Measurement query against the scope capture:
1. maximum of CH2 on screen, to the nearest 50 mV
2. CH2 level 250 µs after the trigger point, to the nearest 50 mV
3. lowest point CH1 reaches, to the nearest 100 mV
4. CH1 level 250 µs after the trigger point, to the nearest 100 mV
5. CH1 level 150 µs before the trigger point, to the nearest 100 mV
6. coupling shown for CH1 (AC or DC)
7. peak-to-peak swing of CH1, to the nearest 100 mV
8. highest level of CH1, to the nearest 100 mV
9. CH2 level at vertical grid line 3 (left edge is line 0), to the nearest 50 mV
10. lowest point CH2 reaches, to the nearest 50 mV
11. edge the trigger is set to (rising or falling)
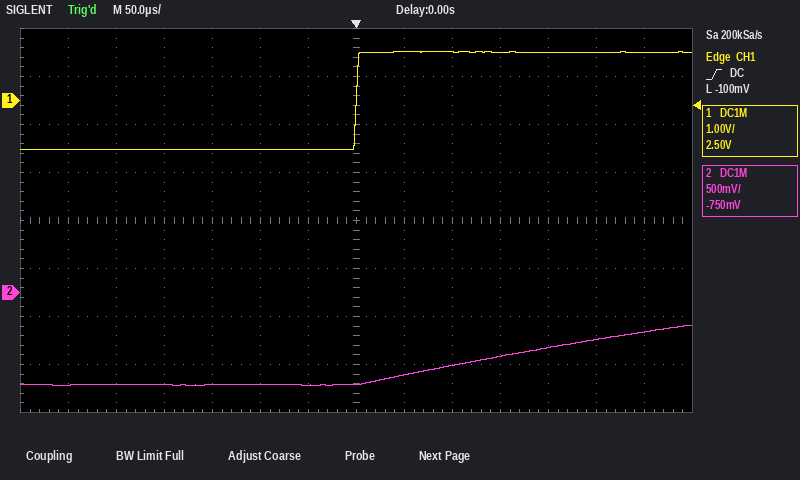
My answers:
-350 mV
-500 mV
-1.0 V
1.0 V
-1.0 V
DC
2.0 V
1.0 V
-950 mV
-950 mV
rising
